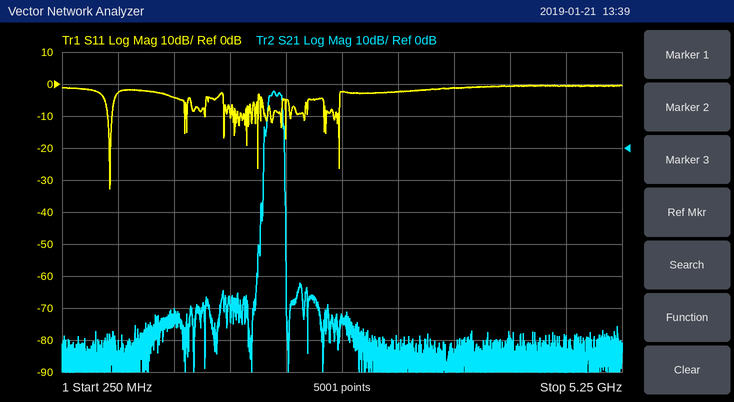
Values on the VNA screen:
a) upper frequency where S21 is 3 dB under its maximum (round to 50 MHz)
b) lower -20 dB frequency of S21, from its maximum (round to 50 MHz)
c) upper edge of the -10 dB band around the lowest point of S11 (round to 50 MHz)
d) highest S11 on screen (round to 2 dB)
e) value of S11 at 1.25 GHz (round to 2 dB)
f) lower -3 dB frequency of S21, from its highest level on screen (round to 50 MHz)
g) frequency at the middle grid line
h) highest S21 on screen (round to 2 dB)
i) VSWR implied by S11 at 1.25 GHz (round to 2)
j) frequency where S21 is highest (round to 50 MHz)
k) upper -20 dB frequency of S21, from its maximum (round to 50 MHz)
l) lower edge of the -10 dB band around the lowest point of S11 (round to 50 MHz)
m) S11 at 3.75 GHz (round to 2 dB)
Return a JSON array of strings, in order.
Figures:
["2.20 GHz", "2.05 GHz", "700 MHz", "0 dB", "-4 dB", "2.10 GHz", "2.75 GHz", "18 dB", "4", "2.15 GHz", "2.25 GHz", "650 MHz", "-2 dB"]
